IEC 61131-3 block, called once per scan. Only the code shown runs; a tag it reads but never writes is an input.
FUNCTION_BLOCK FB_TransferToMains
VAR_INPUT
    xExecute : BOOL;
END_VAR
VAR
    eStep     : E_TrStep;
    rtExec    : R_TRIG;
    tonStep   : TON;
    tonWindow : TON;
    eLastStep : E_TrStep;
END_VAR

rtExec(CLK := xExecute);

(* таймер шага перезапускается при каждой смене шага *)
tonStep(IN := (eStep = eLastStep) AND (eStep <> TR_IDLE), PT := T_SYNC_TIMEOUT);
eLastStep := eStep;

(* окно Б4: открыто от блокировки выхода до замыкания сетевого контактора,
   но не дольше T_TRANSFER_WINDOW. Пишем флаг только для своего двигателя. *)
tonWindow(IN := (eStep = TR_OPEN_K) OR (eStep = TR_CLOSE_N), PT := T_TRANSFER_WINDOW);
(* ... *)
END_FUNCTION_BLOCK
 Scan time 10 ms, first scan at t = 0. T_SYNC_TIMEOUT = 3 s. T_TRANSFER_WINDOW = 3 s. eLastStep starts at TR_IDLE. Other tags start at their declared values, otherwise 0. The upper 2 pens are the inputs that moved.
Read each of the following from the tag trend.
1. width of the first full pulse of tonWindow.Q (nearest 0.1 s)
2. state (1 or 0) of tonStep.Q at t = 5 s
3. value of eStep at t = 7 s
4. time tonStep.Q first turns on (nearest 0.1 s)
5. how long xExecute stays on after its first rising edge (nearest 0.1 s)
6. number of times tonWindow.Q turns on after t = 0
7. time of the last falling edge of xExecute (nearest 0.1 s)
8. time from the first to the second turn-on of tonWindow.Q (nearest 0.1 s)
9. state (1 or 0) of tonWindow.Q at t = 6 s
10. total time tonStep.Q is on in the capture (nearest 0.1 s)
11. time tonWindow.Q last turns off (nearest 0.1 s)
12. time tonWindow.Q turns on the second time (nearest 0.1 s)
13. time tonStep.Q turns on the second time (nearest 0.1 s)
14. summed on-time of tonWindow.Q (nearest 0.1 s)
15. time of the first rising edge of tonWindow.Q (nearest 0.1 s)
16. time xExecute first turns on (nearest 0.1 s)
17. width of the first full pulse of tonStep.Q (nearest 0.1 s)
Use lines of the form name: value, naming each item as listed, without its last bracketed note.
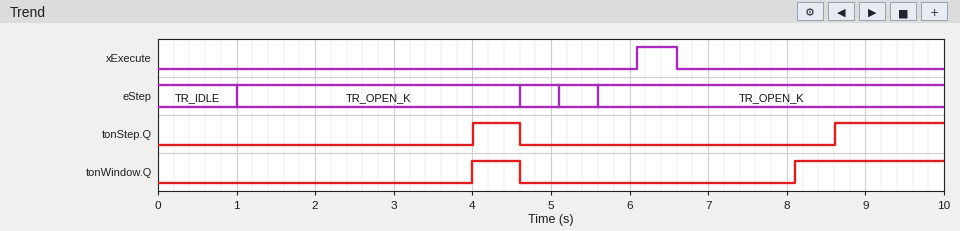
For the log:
width of the first full pulse of tonWindow.Q: 0.6 s
state (1 or 0) of tonStep.Q at t = 5 s: 0
value of eStep at t = 7 s: TR_OPEN_K
time tonStep.Q first turns on: 4.0 s
how long xExecute stays on after its first rising edge: 0.5 s
number of times tonWindow.Q turns on after t = 0: 2
time of the last falling edge of xExecute: 6.6 s
time from the first to the second turn-on of tonWindow.Q: 4.1 s
state (1 or 0) of tonWindow.Q at t = 6 s: 0
total time tonStep.Q is on in the capture: 2.0 s
time tonWindow.Q last turns off: 4.6 s
time tonWindow.Q turns on the second time: 8.1 s
time tonStep.Q turns on the second time: 8.6 s
summed on-time of tonWindow.Q: 2.5 s
time of the first rising edge of tonWindow.Q: 4.0 s
time xExecute first turns on: 6.1 s
width of the first full pulse of tonStep.Q: 0.6 s
